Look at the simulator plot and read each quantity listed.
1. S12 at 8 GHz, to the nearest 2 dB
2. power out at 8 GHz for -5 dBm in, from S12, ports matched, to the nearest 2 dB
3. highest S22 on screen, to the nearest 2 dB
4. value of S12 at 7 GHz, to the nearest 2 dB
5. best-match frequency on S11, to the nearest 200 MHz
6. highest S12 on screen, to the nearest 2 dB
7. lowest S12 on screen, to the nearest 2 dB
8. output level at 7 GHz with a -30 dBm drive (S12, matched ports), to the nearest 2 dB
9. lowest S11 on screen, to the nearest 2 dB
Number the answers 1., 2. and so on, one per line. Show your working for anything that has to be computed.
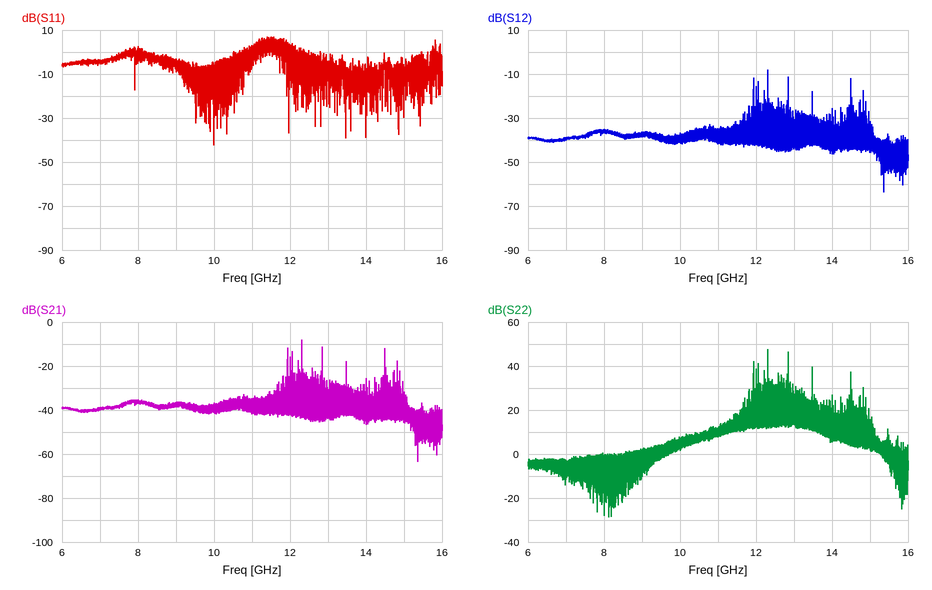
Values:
1. -36 dB
2. -5 dBm + (-36 dB) = -40 dBm
3. 48 dB
4. -40 dB
5. 10.0 GHz
6. -8 dB
7. -64 dB
8. -30 dBm + (-40 dB) = -70 dBm
9. -42 dB
